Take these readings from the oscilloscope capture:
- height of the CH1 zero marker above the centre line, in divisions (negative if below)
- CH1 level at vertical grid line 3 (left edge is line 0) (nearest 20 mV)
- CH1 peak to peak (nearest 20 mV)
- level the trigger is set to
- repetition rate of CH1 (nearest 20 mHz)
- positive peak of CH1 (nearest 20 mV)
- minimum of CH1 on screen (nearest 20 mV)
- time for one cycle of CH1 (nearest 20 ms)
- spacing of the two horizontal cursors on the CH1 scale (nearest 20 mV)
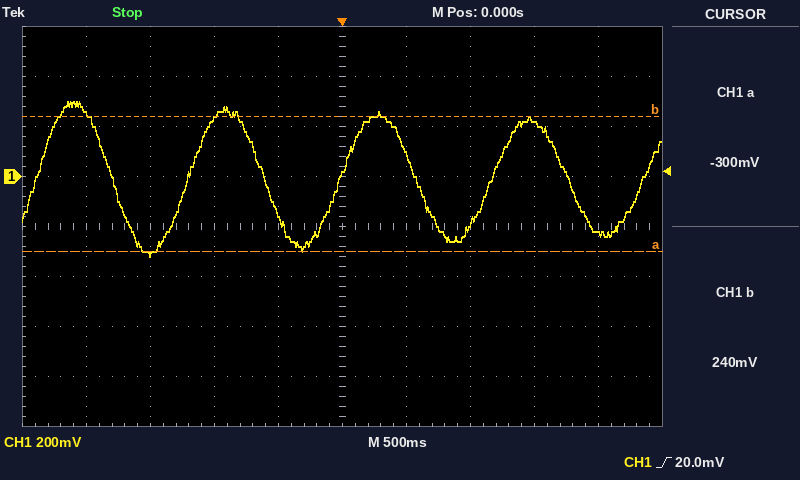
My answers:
+1.0 div
240 mV
620 mV
20.0 mV
840 mHz
300 mV
-320 mV
1.18 s
540 mV
